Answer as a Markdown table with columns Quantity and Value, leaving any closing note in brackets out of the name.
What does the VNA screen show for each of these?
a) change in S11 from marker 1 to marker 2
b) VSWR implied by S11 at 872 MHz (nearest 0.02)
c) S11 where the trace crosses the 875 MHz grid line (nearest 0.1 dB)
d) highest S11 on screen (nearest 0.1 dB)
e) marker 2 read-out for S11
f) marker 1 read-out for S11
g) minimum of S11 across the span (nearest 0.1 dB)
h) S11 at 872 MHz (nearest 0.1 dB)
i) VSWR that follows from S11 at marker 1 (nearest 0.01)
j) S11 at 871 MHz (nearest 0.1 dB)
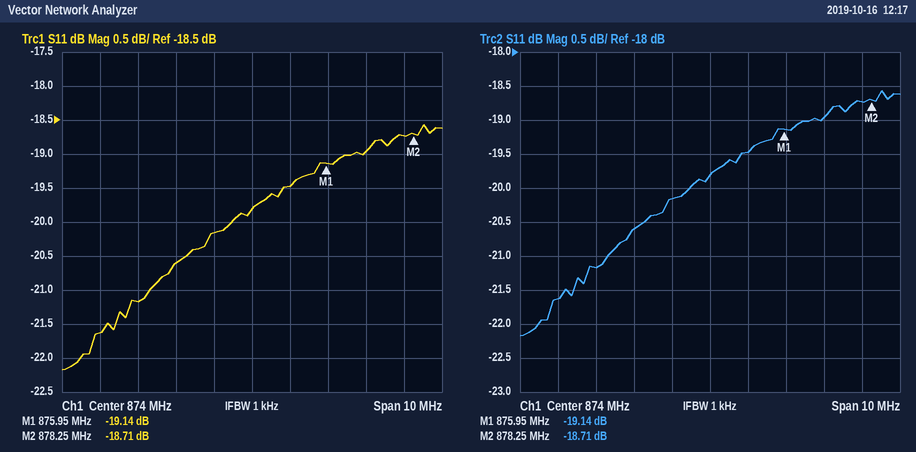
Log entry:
| Quantity | Value |
|---|---|
| change in S11 from marker 1 to marker 2 | 0.43 dB |
| VSWR implied by S11 at 872 MHz | 1.20 |
| S11 where the trace crosses the 875 MHz grid line | -19.5 dB |
| highest S11 on screen | -18.6 dB |
| marker 2 read-out for S11 | -18.71 dB |
| marker 1 read-out for S11 | -19.14 dB |
| minimum of S11 across the span | -22.2 dB |
| S11 at 872 MHz | -20.6 dB |
| VSWR that follows from S11 at marker 1 | 1.25 |
| S11 at 871 MHz | -21.2 dB |
